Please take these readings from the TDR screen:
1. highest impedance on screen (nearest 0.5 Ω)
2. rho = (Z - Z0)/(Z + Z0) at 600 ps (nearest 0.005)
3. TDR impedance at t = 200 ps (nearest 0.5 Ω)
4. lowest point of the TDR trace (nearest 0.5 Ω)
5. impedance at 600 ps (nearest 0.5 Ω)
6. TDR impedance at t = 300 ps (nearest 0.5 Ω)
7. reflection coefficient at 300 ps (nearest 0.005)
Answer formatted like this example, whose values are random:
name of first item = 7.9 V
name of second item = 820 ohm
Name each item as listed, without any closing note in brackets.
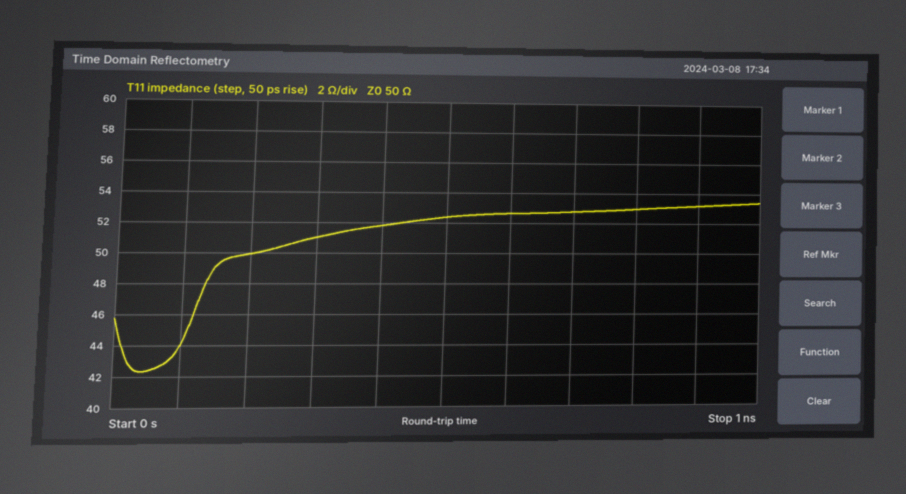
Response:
highest impedance on screen = 53.5 Ω
rho = (Z - Z0)/(Z + Z0) at 600 ps = +0.025
TDR impedance at t = 200 ps = 50.0 Ω
lowest point of the TDR trace = 42.5 Ω
impedance at 600 ps = 52.5 Ω
TDR impedance at t = 300 ps = 51.0 Ω
reflection coefficient at 300 ps = +0.010
